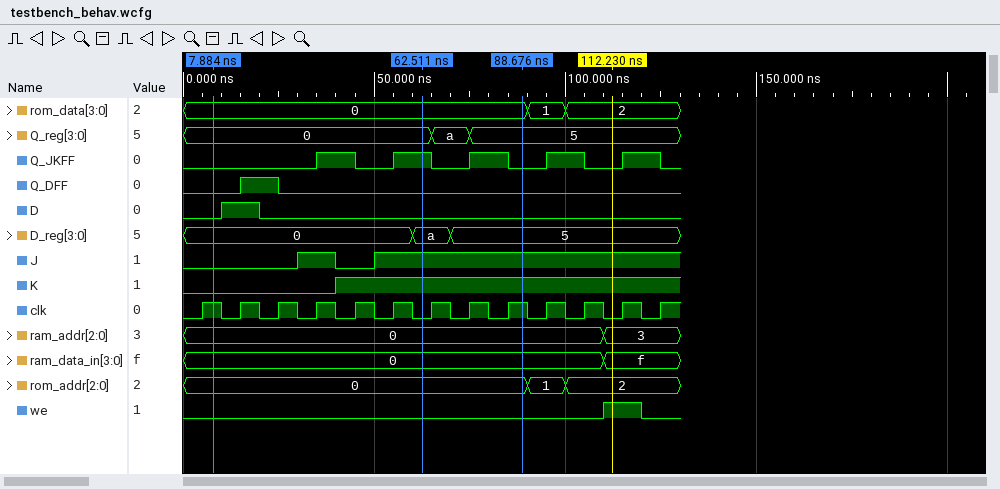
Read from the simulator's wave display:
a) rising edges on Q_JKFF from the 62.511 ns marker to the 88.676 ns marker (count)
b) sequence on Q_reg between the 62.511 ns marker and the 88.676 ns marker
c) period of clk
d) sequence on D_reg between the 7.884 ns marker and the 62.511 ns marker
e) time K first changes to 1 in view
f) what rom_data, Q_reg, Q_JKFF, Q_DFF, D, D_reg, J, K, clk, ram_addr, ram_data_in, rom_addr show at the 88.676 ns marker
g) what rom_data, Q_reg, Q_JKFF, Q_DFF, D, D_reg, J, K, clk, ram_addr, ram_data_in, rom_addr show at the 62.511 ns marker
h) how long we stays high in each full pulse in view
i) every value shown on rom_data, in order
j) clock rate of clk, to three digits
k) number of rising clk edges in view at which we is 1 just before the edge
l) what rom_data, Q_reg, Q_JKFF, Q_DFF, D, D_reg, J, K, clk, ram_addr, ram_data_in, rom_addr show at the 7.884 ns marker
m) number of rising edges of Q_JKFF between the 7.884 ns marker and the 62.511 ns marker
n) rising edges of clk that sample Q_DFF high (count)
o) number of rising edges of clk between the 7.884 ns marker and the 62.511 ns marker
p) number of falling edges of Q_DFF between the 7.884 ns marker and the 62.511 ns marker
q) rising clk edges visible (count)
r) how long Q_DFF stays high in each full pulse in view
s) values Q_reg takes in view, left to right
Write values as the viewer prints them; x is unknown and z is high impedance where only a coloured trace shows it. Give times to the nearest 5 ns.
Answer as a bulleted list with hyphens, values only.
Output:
- 1
- 0, a, 5
- 10 ns
- 0, a
- 40 ns
- rom_data=0, Q_reg=5, Q_JKFF=0, Q_DFF=0, D=0, D_reg=5, J=1, K=1, clk=1, ram_addr=0, ram_data_in=0, rom_addr=0
- rom_data=0, Q_reg=0, Q_JKFF=1, Q_DFF=0, D=0, D_reg=a, J=1, K=1, clk=0, ram_addr=0, ram_data_in=0, rom_addr=0
- 10 ns
- 0, 1, 2
- 100 MHz
- 1
- rom_data=0, Q_reg=0, Q_JKFF=0, Q_DFF=0, D=0, D_reg=0, J=0, K=0, clk=1, ram_addr=0, ram_data_in=0, rom_addr=0
- 2
- 1
- 5
- 1
- 13
- 10 ns
- 0, a, 5
